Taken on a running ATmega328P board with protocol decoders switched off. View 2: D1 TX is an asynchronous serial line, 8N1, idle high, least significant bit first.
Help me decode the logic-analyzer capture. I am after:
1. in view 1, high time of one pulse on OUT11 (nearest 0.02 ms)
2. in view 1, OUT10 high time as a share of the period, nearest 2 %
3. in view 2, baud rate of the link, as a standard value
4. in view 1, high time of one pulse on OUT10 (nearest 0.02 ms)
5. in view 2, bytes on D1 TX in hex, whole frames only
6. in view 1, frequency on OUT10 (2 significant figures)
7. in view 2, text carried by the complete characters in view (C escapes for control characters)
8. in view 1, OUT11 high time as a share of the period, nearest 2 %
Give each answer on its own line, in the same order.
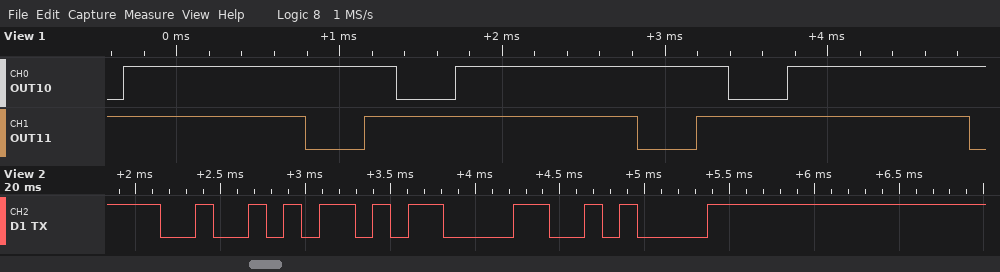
1.68 ms
82 %
9600 baud
1.68 ms
52 0D 0A
490 Hz
"R\r\n"
82 %
